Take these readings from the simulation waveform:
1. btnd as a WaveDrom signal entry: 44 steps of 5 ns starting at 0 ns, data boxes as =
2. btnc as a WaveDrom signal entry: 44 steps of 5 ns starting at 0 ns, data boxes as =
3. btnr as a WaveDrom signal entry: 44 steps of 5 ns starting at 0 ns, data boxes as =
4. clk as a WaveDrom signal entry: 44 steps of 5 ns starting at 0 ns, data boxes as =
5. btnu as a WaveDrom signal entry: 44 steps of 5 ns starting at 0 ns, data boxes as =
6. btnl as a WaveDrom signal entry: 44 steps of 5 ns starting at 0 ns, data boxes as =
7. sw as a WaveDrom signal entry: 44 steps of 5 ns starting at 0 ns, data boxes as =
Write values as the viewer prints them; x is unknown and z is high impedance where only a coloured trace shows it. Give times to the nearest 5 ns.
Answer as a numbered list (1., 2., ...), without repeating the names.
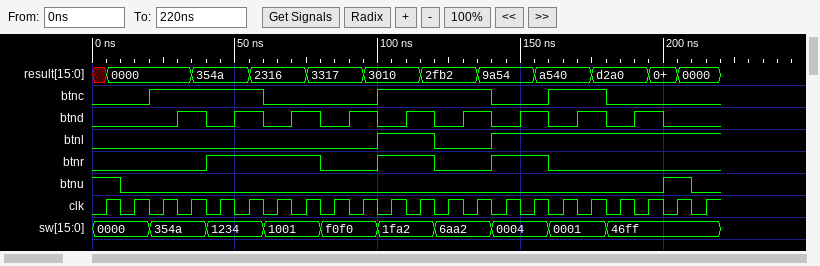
1. {name: 'btnd', wave: '0.....1.0.1.0.1.0.1.0.1.0.1.0.1.0.1.0.1.0...'}
2. {name: 'btnc', wave: '0...1.......0.......1.......0...1...0.......'}
3. {name: 'btnr', wave: '0.......1.......0...1...0...1...0...........'}
4. {name: 'clk', wave: '01010101010101010101010101010101010101010101'}
5. {name: 'btnu', wave: '1.0.....................................1.0.'}
6. {name: 'btnl', wave: '0...................1...0...1...............'}
7. {name: 'sw', wave: '=...=...=...=...=...=...=...=...=...=.......', data: '0000 354a 1234 1001 f0f0 1fa2 6aa2 0004 0001 46ff'}
